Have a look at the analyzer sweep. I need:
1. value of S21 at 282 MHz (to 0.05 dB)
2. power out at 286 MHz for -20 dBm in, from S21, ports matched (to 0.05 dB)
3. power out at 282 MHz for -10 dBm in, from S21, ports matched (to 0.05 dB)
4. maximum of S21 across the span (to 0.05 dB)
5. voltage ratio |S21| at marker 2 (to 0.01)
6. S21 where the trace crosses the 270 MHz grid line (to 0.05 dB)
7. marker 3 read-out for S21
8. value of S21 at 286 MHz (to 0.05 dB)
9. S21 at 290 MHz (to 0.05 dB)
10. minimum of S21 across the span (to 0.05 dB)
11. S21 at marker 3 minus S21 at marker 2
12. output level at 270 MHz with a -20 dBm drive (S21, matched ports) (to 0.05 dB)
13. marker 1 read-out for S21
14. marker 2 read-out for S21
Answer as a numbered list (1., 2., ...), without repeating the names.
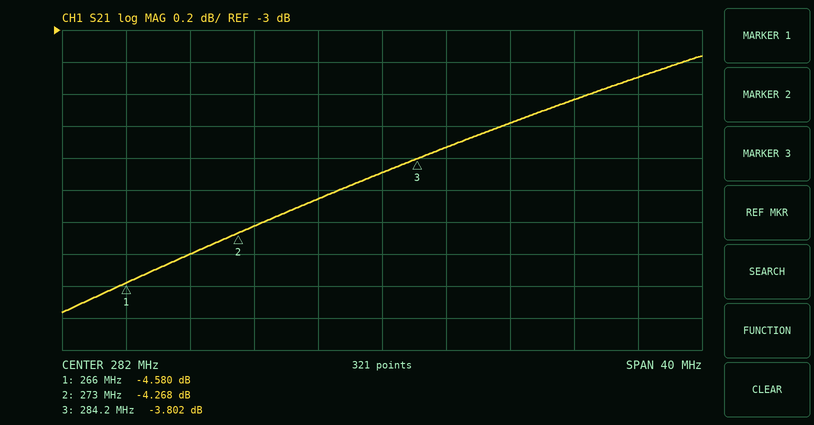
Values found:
1. -3.90 dB
2. -23.75 dBm
3. -13.90 dBm
4. -3.15 dB
5. 0.61
6. -4.40 dB
7. -3.802 dB
8. -3.75 dB
9. -3.60 dB
10. -4.75 dB
11. 0.466 dB
12. -24.40 dBm
13. -4.580 dB
14. -4.268 dB
